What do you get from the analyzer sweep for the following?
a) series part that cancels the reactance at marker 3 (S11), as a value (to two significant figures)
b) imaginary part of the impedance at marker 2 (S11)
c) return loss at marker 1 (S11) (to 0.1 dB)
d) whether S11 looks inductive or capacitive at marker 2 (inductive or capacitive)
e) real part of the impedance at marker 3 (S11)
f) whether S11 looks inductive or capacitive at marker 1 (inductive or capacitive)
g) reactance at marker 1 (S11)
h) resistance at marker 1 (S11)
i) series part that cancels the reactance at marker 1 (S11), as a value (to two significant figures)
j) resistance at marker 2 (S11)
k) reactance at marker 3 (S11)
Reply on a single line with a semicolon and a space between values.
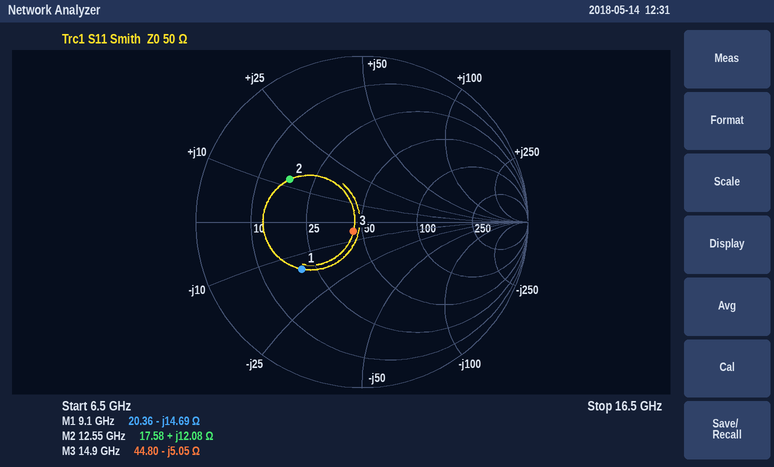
54 pH; +12.08 Ω; 6.7 dB; inductive; 44.80 Ω; capacitive; -14.69 Ω; 20.36 Ω; 260 pH; 17.58 Ω; -5.05 Ω
